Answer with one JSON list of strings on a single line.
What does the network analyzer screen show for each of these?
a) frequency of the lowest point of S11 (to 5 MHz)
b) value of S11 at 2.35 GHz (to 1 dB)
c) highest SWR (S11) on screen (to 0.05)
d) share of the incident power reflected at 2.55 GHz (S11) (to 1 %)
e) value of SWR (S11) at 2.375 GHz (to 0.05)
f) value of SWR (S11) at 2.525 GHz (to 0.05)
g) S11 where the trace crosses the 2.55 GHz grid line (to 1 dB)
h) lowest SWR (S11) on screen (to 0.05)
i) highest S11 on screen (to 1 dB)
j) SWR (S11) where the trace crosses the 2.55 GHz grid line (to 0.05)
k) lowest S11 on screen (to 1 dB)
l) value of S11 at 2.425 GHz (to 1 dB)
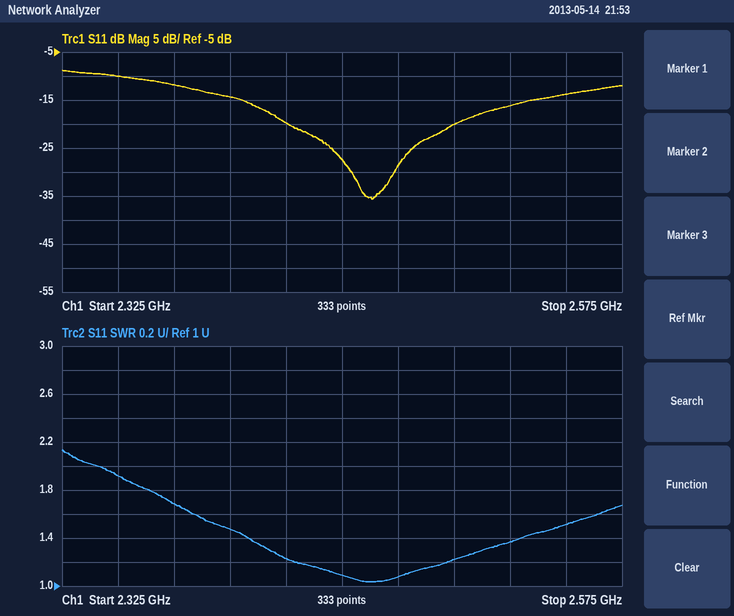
["2.465 GHz", "-10 dB", "2.15", "4 %", "1.70", "1.35", "-14 dB", "1.05", "-9 dB", "1.50", "-36 dB", "-20 dB"]
